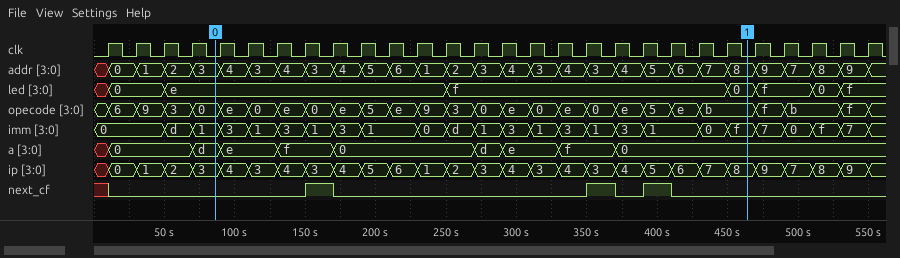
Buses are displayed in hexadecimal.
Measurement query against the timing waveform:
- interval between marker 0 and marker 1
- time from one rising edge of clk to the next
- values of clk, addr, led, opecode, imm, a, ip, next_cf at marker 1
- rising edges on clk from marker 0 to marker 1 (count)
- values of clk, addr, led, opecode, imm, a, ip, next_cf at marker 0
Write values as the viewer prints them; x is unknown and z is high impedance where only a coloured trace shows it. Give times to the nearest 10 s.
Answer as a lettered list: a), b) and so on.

a) 380 s
b) 20 s
c) clk=0, addr=8, led=0, opecode=b, imm=f, a=0, ip=8, next_cf=0
d) 19
e) clk=0, addr=3, led=e, opecode=0, imm=1, a=d, ip=3, next_cf=0
